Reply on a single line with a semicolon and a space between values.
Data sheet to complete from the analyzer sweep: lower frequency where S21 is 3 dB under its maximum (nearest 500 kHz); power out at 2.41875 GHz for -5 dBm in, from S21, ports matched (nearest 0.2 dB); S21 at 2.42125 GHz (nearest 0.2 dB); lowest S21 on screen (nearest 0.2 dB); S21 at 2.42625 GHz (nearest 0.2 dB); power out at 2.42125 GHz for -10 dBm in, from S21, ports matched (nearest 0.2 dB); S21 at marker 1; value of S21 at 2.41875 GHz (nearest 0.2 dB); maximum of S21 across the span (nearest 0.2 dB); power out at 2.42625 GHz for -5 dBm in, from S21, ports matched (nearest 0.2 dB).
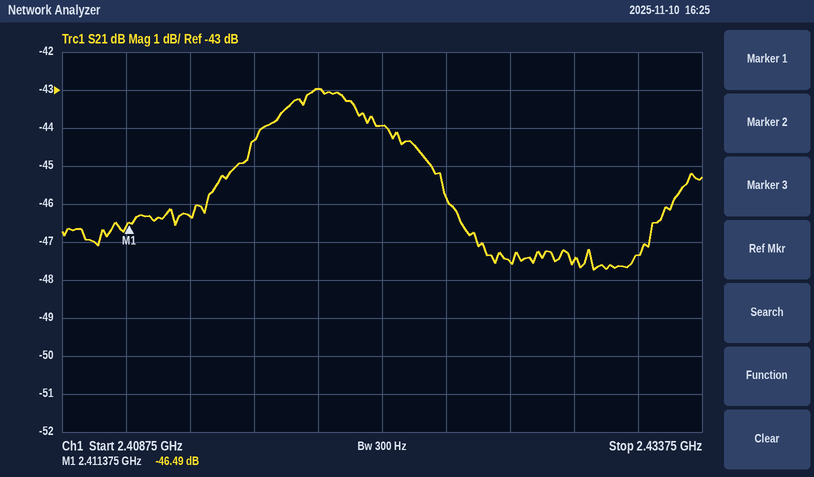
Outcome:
2.4145 GHz; -48.0 dBm; -44.0 dB; -47.8 dB; -47.6 dB; -54.0 dBm; -46.49 dB; -43.0 dB; -43.0 dB; -52.6 dBm
